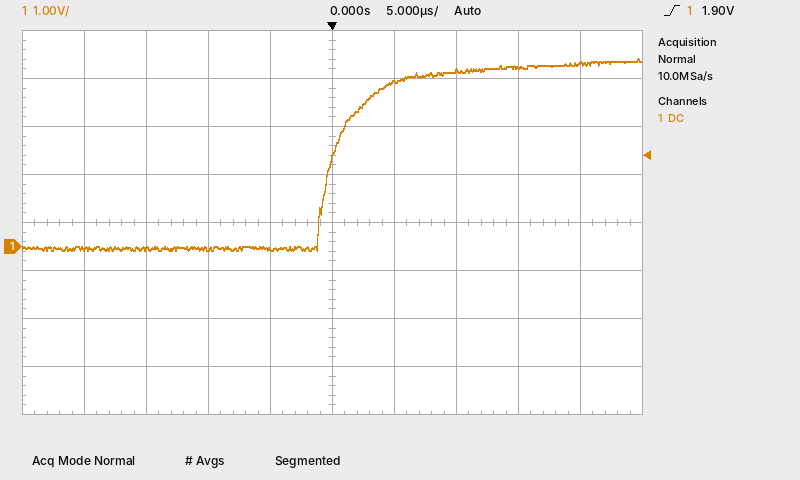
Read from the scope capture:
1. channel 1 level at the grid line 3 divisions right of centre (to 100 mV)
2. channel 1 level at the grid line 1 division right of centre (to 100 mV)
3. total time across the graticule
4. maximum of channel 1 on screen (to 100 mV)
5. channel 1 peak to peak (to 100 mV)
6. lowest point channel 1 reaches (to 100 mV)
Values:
3.7 V
3.4 V
50 µs
3.9 V
4.0 V
-100 mV
